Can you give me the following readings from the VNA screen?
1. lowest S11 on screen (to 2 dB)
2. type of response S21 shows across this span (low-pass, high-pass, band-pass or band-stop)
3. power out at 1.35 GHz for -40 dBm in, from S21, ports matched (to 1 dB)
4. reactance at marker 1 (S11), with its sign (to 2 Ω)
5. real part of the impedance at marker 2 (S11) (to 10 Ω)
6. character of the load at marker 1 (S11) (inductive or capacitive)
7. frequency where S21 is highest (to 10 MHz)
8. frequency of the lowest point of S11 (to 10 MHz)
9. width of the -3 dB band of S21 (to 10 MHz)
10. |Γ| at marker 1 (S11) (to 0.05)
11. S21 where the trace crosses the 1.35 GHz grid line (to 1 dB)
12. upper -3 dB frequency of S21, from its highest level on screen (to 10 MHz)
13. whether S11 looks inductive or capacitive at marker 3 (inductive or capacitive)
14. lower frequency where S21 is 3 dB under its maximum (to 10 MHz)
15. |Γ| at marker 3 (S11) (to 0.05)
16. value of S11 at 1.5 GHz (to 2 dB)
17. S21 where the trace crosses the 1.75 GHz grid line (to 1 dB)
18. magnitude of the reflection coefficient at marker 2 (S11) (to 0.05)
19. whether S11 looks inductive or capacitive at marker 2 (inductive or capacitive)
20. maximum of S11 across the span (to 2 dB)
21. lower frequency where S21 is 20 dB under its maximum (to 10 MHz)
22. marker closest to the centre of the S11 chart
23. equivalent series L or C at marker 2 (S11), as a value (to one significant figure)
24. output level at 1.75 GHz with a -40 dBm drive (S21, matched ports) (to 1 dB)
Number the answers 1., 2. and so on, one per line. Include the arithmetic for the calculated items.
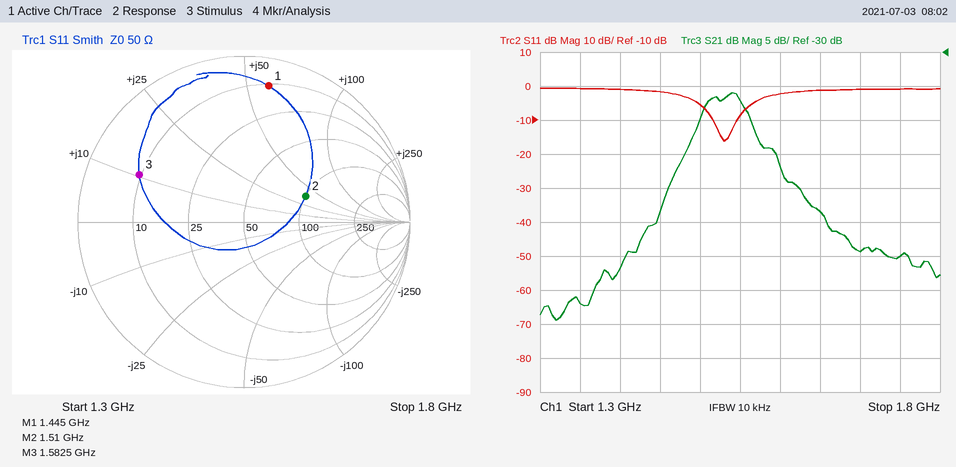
1. -16 dB
2. band-pass
3. -40 dBm + (-67 dB) = -107 dBm
4. +58 Ω
5. 100 Ω
6. inductive
7. 1.54 GHz
8. 1.53 GHz
9. 1.56 GHz − 1.50 GHz = 60 MHz
10. 0.85
11. -67 dB
12. 1.56 GHz
13. inductive
14. 1.50 GHz
15. 0.70
16. -6 dB
17. -60 dB
18. 0.40
19. inductive
20. 0 dB
21. 1.43 GHz
22. marker 2
23. L = 40 Ω/(2π × 1.51 GHz) ≈ 4 nH
24. -40 dBm + (-60 dB) = -100 dBm
